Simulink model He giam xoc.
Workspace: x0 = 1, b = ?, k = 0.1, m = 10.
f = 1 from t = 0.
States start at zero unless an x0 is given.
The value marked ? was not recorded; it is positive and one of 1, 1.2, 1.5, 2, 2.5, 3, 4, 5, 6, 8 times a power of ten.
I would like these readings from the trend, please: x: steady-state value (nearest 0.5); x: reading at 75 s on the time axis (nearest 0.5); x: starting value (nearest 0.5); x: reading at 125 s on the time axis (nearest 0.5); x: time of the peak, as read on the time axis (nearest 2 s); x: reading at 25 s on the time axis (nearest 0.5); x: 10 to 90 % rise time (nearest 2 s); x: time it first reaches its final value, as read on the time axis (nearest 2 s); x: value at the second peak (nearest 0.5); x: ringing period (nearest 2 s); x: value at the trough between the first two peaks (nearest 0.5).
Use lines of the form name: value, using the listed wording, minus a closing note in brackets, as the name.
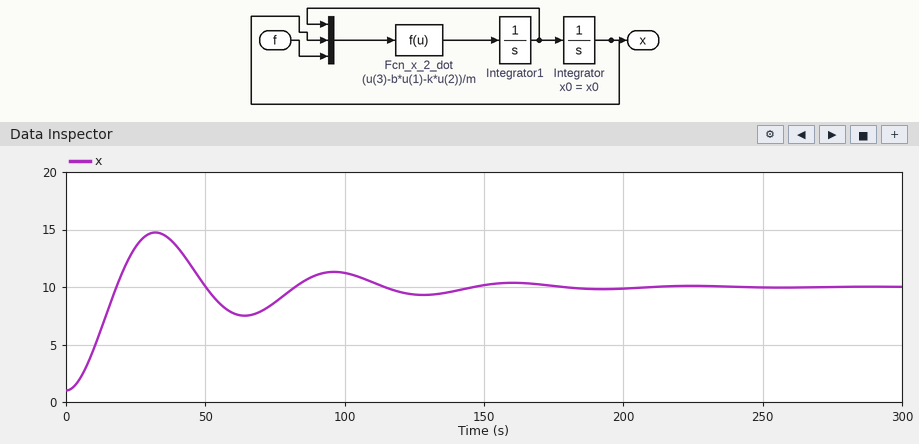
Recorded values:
x: steady-state value: 10.0
x: reading at 75 s on the time axis: 8.5
x: starting value: 1.0
x: reading at 125 s on the time axis: 9.5
x: time of the peak, as read on the time axis: 32 s
x: reading at 25 s on the time axis: 13.5
x: 10 to 90 % rise time: 12 s
x: time it first reaches its final value, as read on the time axis: 18 s
x: value at the second peak: 11.5
x: ringing period: 64 s
x: value at the trough between the first two peaks: 7.5
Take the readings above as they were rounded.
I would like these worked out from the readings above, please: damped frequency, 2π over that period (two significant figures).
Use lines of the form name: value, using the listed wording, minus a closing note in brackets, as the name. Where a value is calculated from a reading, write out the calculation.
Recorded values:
damped frequency, 2π over that period: 2π / 64 = 0.098 rad/s
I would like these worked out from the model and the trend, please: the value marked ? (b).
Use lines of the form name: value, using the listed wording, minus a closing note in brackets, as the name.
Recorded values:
the value marked ?: 0.4
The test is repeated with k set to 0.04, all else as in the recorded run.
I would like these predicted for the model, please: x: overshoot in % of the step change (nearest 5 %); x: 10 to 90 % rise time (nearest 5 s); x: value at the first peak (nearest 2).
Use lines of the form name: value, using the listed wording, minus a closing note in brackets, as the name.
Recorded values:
x: overshoot in % of the step change: 35 %
x: 10 to 90 % rise time: 20 s
x: value at the first peak: 34
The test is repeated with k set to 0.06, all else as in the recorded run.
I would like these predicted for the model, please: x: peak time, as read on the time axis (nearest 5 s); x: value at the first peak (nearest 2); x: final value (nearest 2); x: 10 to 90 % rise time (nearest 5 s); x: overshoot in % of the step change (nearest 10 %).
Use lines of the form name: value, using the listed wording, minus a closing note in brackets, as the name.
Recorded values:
x: peak time, as read on the time axis: 40 s
x: value at the first peak: 24
x: final value: 16
x: 10 to 90 % rise time: 15 s
x: overshoot in % of the step change: 40 %
